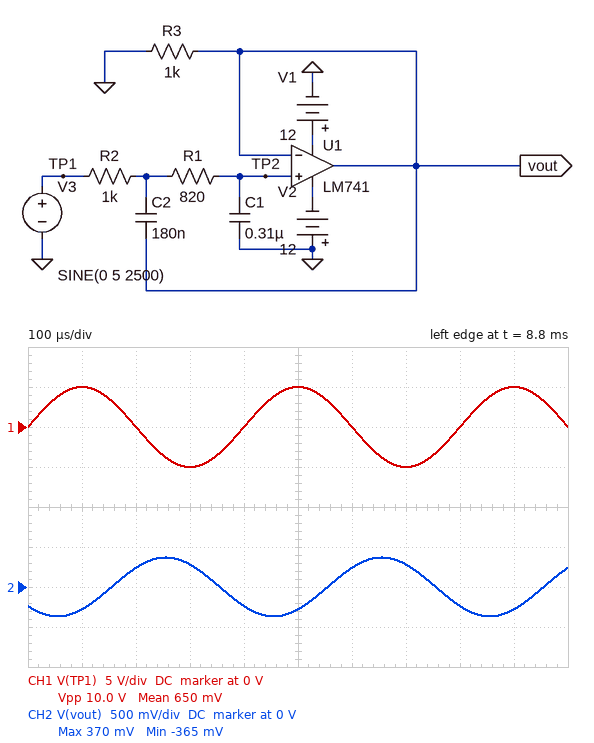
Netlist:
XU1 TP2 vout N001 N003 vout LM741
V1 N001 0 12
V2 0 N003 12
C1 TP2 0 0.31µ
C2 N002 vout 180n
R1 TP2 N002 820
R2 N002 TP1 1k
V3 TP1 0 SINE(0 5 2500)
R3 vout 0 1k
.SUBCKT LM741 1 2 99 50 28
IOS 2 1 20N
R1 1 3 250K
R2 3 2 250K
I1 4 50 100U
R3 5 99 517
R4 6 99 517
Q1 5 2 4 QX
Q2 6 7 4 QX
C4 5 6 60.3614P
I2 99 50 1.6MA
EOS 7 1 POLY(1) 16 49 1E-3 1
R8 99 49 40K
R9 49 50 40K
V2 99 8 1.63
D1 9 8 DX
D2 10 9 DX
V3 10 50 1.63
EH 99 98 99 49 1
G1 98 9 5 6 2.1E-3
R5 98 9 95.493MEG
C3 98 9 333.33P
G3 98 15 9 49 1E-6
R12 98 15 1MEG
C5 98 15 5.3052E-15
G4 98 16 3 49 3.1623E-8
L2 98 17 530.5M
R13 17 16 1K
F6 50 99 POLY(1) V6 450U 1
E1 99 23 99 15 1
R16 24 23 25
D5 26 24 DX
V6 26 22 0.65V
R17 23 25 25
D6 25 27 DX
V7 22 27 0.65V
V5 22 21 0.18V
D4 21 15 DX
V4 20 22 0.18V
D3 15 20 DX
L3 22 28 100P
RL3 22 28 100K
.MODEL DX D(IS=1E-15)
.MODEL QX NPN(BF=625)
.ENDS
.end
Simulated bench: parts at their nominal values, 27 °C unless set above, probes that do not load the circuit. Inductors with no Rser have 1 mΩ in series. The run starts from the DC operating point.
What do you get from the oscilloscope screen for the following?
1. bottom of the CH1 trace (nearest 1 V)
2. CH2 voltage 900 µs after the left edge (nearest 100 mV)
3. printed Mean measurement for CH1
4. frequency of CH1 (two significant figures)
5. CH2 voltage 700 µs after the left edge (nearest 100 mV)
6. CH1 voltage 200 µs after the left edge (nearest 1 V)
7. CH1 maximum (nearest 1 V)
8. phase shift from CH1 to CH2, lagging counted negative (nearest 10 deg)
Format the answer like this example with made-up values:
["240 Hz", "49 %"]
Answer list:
["-5 V", "-300 mV", "650 mV", "2.5 kHz", "300 mV", "0 V", "5 V", "-140 deg"]
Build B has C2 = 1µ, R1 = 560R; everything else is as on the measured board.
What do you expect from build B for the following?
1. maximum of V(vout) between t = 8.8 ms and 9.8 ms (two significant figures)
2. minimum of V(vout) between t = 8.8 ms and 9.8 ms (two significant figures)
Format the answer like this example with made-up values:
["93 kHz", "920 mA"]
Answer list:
["120 mV", "-120 mV"]
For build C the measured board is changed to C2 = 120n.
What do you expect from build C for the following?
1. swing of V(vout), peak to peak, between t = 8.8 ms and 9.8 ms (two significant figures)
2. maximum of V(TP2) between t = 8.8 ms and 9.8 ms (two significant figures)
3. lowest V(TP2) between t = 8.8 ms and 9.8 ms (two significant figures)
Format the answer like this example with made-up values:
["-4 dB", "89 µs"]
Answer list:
["910 mV", "450 mV", "-450 mV"]
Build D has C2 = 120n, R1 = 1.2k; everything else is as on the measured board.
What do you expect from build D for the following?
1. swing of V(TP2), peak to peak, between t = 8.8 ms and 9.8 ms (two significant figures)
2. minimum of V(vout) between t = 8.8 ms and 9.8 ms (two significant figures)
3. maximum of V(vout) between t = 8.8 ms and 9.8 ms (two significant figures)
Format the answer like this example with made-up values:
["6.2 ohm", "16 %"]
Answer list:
["680 mV", "-340 mV", "340 mV"]
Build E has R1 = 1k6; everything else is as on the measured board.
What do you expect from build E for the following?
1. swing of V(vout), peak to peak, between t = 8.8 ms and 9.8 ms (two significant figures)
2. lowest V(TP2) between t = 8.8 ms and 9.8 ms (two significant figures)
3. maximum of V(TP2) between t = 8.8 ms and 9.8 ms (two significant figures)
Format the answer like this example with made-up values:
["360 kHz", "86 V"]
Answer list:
["410 mV", "-200 mV", "200 mV"]
